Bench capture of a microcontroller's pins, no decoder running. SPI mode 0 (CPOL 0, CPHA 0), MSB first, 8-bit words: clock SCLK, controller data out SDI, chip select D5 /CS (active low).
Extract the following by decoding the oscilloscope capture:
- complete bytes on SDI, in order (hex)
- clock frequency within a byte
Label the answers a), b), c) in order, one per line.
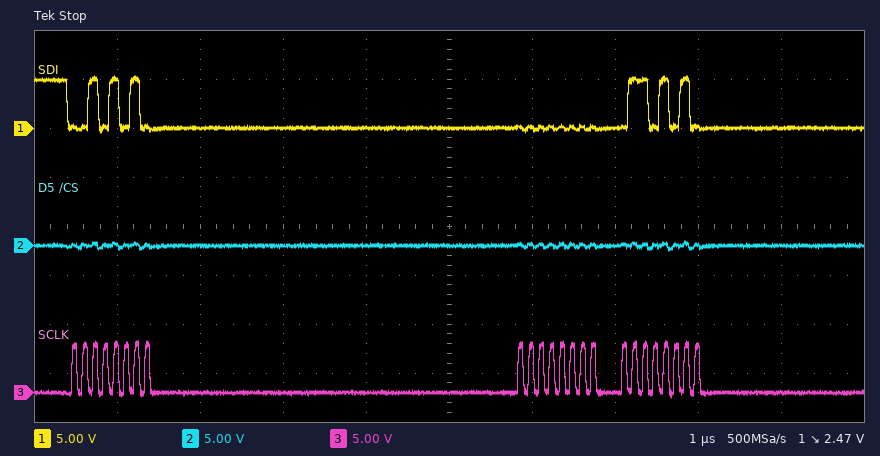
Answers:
a) 2A 00 6A
b) 8 MHz
